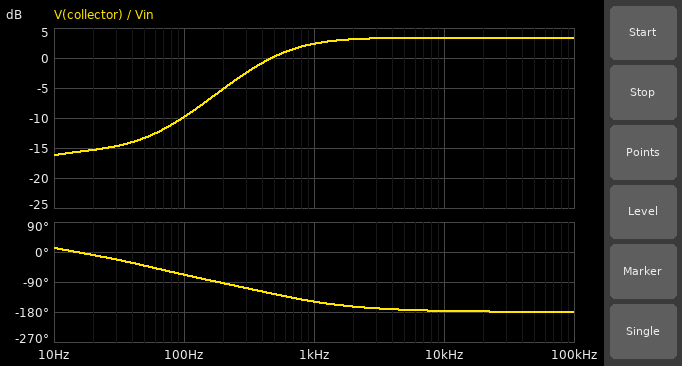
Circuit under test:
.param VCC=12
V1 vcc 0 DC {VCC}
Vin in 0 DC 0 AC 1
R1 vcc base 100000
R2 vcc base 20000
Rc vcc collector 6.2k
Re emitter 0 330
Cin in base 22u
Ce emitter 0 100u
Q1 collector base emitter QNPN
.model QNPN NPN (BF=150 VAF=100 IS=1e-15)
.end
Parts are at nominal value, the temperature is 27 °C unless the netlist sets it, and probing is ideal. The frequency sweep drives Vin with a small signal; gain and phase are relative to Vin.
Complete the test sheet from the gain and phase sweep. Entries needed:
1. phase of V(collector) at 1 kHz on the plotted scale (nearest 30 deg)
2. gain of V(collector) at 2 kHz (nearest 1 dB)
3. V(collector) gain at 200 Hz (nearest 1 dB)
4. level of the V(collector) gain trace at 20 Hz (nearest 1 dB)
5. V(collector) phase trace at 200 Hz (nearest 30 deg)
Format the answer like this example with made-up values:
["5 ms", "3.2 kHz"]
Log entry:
["-150 deg", "3 dB", "-5 dB", "-15 dB", "-90 deg"]
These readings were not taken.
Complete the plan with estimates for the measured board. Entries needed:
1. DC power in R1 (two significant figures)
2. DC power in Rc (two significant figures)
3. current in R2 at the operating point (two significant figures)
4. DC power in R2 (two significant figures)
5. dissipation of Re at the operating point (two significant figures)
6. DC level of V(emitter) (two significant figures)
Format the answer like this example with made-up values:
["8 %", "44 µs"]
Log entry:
["1.1 mW", "20 mW", "520 µA", "5.5 mW", "1.9 mW", "800 mV"]
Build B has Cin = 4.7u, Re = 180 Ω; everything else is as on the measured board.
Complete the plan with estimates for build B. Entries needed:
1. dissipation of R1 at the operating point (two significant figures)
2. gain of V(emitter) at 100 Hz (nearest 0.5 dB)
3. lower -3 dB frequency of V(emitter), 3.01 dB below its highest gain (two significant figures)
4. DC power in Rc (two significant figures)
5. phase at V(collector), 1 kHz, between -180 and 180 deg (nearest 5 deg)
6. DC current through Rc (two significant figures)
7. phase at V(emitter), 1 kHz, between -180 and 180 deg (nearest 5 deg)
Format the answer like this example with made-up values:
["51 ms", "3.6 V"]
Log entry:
["1.2 mW", "-27.0 dB", "8.7 Hz", "21 mW", "-110 deg", "1.9 mA", "-25 deg"]
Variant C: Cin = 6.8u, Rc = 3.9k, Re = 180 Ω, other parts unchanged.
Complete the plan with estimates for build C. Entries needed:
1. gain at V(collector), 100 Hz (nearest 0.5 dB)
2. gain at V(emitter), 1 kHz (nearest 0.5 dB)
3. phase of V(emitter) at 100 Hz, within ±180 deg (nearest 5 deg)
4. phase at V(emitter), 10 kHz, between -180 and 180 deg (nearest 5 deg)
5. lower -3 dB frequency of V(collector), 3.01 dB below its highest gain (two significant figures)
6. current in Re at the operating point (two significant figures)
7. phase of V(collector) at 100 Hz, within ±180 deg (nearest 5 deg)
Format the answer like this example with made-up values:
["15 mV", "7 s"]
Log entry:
["-18.0 dB", "-25.0 dB", "0 deg", "-80 deg", "2.0 kHz", "3.5 mA", "-65 deg"]
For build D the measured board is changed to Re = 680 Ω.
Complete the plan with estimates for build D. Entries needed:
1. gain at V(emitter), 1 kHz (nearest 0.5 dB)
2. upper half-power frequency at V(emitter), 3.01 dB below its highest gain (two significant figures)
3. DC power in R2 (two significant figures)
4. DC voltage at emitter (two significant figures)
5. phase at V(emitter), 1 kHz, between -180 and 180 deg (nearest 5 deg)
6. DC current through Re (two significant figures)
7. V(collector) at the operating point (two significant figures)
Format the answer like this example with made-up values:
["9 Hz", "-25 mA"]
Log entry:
["-22.0 dB", "490 Hz", "4.7 mW", "1.5 V", "-65 deg", "2.3 mA", "1.6 V"]
